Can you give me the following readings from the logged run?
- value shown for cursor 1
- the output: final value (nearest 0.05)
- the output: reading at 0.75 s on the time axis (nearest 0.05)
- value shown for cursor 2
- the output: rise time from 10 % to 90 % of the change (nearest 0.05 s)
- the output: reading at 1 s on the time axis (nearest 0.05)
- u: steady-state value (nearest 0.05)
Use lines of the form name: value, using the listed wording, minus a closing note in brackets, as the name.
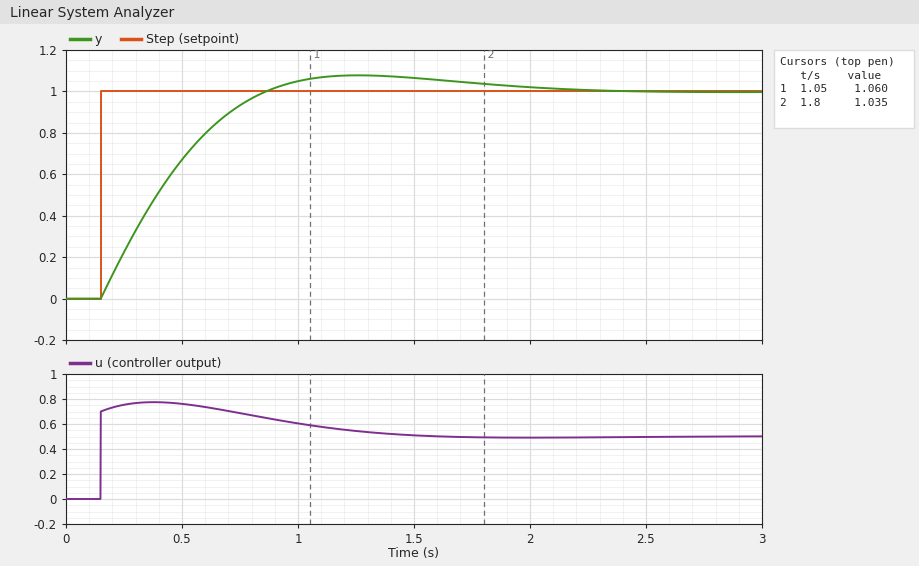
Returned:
value shown for cursor 1: 1.060
the output: final value: 1.00
the output: reading at 0.75 s on the time axis: 0.95
value shown for cursor 2: 1.035
the output: rise time from 10 % to 90 % of the change: 0.50 s
the output: reading at 1 s on the time axis: 1.05
u: steady-state value: 0.50
